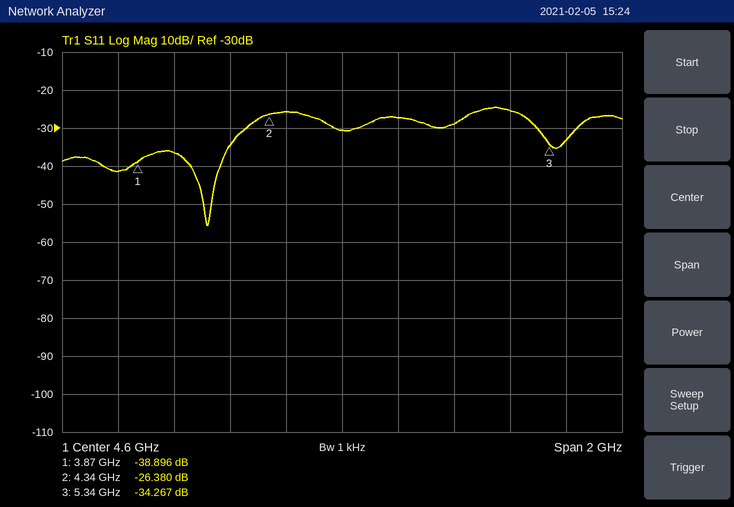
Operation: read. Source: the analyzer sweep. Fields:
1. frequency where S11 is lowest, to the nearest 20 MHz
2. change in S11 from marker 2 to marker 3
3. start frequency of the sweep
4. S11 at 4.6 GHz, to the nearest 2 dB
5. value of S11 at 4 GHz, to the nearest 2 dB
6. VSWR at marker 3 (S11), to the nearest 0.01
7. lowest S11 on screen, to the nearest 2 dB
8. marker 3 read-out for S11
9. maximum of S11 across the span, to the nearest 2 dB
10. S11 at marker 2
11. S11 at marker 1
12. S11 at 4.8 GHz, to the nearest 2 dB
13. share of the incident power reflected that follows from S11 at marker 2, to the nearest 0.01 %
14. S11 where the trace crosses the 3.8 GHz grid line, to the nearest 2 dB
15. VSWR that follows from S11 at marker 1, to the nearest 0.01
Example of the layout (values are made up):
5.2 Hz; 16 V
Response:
4.12 GHz; -7.887 dB; 3.6 GHz; -30 dB; -36 dB; 1.04; -56 dB; -34.267 dB; -24 dB; -26.380 dB; -38.896 dB; -28 dB; 0.23 %; -42 dB; 1.02
